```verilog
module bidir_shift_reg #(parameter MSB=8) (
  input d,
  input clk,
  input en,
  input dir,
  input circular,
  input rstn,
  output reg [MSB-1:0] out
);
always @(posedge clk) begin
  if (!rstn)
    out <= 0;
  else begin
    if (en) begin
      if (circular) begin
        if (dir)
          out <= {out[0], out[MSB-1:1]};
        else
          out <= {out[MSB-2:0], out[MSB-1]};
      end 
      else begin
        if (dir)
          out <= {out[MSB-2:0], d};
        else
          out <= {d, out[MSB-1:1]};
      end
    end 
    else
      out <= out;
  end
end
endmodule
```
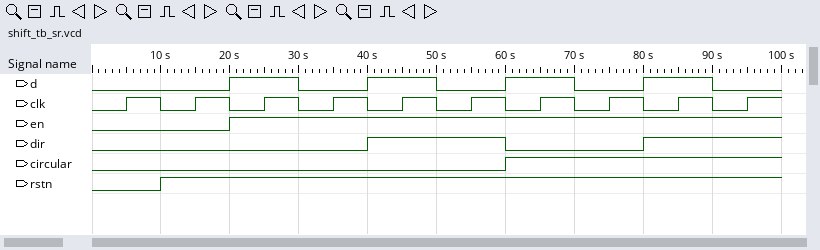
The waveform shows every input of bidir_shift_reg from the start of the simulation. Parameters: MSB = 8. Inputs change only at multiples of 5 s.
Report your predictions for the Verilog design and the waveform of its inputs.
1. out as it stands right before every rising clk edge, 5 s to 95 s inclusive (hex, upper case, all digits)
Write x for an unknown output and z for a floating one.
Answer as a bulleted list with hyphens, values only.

- x, 00, 00, 80, 40, 81, 02, 04, 08, 04
